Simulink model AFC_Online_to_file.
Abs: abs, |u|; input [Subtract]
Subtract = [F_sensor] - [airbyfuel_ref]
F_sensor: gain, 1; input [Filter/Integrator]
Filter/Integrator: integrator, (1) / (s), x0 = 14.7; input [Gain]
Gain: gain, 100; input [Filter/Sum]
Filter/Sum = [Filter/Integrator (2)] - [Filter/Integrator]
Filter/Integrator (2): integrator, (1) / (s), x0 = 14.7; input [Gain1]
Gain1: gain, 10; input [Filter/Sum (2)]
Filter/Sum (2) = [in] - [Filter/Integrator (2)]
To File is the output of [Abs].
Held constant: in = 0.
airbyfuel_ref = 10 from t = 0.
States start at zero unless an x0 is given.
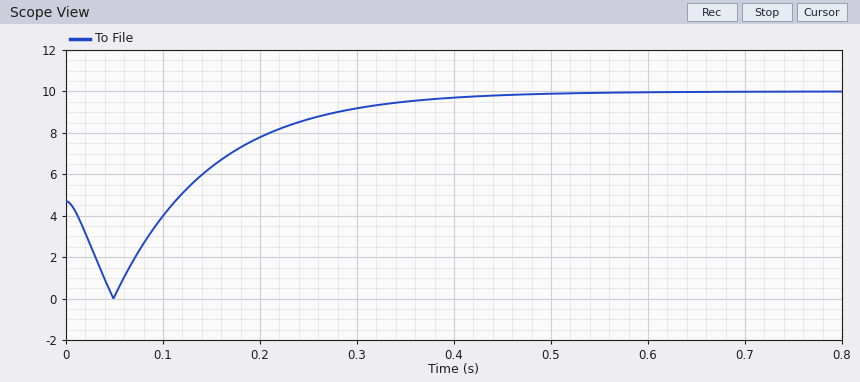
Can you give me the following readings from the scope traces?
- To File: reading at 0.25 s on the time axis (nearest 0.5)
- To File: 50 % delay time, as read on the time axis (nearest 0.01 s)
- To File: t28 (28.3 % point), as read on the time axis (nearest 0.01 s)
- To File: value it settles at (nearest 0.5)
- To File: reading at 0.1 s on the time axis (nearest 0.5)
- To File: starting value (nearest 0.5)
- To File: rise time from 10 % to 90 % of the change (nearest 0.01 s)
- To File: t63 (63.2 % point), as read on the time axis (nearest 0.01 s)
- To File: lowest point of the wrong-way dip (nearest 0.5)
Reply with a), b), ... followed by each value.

a) 8.5
b) 0.18 s
c) 0.15 s
d) 10.0
e) 4.0
f) 4.5
g) 0.22 s
h) 0.21 s
i) 0.0
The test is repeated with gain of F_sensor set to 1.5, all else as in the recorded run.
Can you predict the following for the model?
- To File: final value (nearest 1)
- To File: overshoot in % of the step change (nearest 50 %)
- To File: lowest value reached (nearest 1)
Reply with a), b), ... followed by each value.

a) 10
b) 500 %
c) 0
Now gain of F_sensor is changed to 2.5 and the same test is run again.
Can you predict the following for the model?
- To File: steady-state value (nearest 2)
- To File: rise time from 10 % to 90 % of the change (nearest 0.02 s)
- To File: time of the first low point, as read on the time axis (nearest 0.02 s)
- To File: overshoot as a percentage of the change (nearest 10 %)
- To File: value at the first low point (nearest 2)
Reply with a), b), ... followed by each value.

a) 10
b) 0.06 s
c) 0.14 s
d) 60 %
e) 0
